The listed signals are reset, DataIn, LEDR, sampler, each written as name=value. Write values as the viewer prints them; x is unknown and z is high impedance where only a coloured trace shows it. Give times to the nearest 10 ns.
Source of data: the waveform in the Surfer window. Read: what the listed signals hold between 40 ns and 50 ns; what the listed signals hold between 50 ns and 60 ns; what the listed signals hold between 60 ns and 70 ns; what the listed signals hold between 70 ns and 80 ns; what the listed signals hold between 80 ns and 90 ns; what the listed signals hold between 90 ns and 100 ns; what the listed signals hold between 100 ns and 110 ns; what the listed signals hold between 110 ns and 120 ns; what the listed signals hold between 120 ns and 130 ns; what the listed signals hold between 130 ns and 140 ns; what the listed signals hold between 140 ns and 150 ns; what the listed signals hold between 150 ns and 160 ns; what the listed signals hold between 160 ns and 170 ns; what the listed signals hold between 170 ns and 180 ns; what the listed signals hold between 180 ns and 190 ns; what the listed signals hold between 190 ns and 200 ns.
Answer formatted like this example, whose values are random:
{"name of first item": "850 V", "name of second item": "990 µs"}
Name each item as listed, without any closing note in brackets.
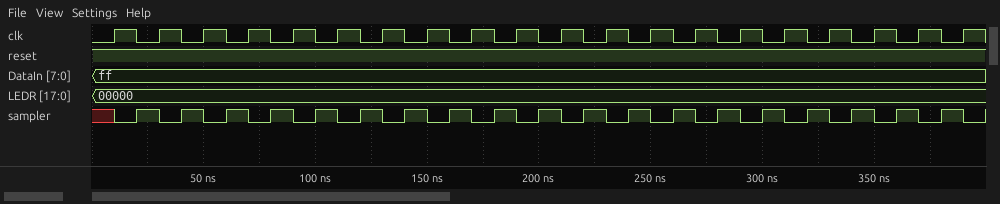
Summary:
{"what the listed signals hold between 40 ns and 50 ns": "reset=1, DataIn=ff, LEDR=00000, sampler=1", "what the listed signals hold between 50 ns and 60 ns": "reset=1, DataIn=ff, LEDR=00000, sampler=0", "what the listed signals hold between 60 ns and 70 ns": "reset=1, DataIn=ff, LEDR=00000, sampler=1", "what the listed signals hold between 70 ns and 80 ns": "reset=1, DataIn=ff, LEDR=00000, sampler=0", "what the listed signals hold between 80 ns and 90 ns": "reset=1, DataIn=ff, LEDR=00000, sampler=1", "what the listed signals hold between 90 ns and 100 ns": "reset=1, DataIn=ff, LEDR=00000, sampler=0", "what the listed signals hold between 100 ns and 110 ns": "reset=1, DataIn=ff, LEDR=00000, sampler=1", "what the listed signals hold between 110 ns and 120 ns": "reset=1, DataIn=ff, LEDR=00000, sampler=0", "what the listed signals hold between 120 ns and 130 ns": "reset=1, DataIn=ff, LEDR=00000, sampler=1", "what the listed signals hold between 130 ns and 140 ns": "reset=1, DataIn=ff, LEDR=00000, sampler=0", "what the listed signals hold between 140 ns and 150 ns": "reset=1, DataIn=ff, LEDR=00000, sampler=1", "what the listed signals hold between 150 ns and 160 ns": "reset=1, DataIn=ff, LEDR=00000, sampler=0", "what the listed signals hold between 160 ns and 170 ns": "reset=1, DataIn=ff, LEDR=00000, sampler=1", "what the listed signals hold between 170 ns and 180 ns": "reset=1, DataIn=ff, LEDR=00000, sampler=0", "what the listed signals hold between 180 ns and 190 ns": "reset=1, DataIn=ff, LEDR=00000, sampler=1", "what the listed signals hold between 190 ns and 200 ns": "reset=1, DataIn=ff, LEDR=00000, sampler=0"}
